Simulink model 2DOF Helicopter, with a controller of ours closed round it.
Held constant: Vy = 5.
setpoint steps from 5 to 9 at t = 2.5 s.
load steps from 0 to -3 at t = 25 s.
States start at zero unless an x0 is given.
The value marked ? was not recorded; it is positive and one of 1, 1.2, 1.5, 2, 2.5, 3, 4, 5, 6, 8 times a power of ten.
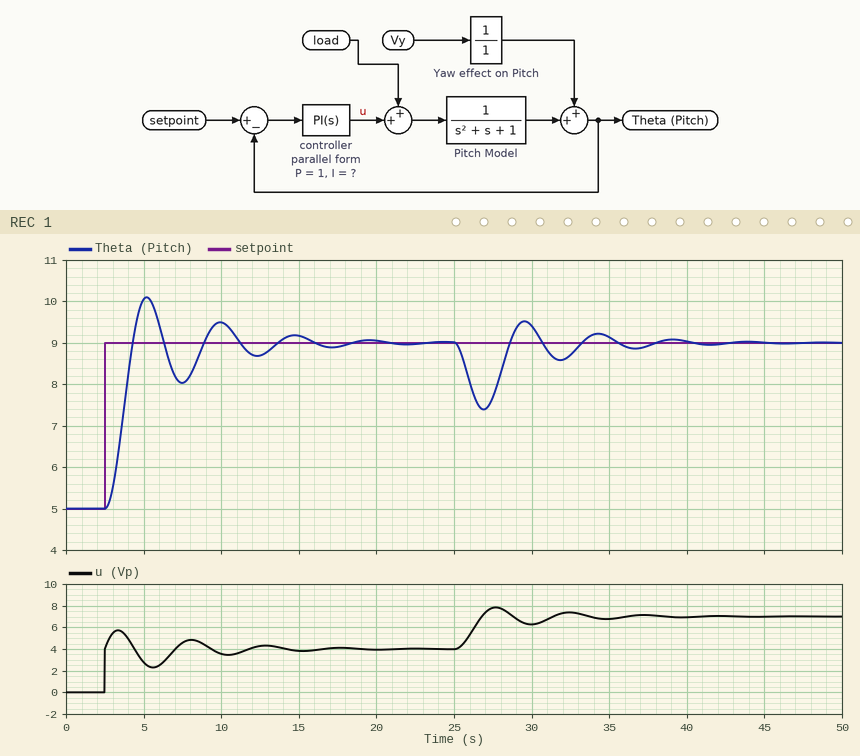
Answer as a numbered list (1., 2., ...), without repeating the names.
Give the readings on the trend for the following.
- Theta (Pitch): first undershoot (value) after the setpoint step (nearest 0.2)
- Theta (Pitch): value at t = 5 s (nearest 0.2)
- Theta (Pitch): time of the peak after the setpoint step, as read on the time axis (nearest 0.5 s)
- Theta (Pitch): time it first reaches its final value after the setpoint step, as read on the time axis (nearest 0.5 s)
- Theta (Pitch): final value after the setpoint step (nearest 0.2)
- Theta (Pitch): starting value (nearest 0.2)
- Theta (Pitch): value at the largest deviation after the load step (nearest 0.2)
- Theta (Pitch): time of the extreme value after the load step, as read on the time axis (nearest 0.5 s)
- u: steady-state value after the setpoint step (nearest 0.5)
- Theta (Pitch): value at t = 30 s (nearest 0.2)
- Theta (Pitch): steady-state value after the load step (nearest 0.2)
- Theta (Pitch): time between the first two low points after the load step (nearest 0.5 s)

1. 8.0
2. 10.0
3. 5.0 s
4. 4.5 s
5. 9.0
6. 5.0
7. 7.4
8. 27.0 s
9. 4.0
10. 9.4
11. 9.0
12. 5.0 s
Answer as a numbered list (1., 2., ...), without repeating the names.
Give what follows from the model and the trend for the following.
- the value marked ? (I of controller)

1. 1
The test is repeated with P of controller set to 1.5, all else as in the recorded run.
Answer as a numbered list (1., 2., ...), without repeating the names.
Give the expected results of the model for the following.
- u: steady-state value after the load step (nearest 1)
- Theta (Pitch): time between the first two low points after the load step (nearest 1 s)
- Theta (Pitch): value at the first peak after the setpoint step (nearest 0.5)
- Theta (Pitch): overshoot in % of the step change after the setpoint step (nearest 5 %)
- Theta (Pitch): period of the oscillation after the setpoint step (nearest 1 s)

1. 7
2. 4 s
3. 10.0
4. 25 %
5. 4 s
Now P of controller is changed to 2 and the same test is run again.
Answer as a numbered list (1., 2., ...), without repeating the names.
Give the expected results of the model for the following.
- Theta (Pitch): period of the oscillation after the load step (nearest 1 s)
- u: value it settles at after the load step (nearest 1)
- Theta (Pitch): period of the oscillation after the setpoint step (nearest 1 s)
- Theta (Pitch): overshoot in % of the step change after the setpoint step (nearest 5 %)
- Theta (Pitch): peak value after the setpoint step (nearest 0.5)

1. 4 s
2. 7
3. 4 s
4. 25 %
5. 10.0
